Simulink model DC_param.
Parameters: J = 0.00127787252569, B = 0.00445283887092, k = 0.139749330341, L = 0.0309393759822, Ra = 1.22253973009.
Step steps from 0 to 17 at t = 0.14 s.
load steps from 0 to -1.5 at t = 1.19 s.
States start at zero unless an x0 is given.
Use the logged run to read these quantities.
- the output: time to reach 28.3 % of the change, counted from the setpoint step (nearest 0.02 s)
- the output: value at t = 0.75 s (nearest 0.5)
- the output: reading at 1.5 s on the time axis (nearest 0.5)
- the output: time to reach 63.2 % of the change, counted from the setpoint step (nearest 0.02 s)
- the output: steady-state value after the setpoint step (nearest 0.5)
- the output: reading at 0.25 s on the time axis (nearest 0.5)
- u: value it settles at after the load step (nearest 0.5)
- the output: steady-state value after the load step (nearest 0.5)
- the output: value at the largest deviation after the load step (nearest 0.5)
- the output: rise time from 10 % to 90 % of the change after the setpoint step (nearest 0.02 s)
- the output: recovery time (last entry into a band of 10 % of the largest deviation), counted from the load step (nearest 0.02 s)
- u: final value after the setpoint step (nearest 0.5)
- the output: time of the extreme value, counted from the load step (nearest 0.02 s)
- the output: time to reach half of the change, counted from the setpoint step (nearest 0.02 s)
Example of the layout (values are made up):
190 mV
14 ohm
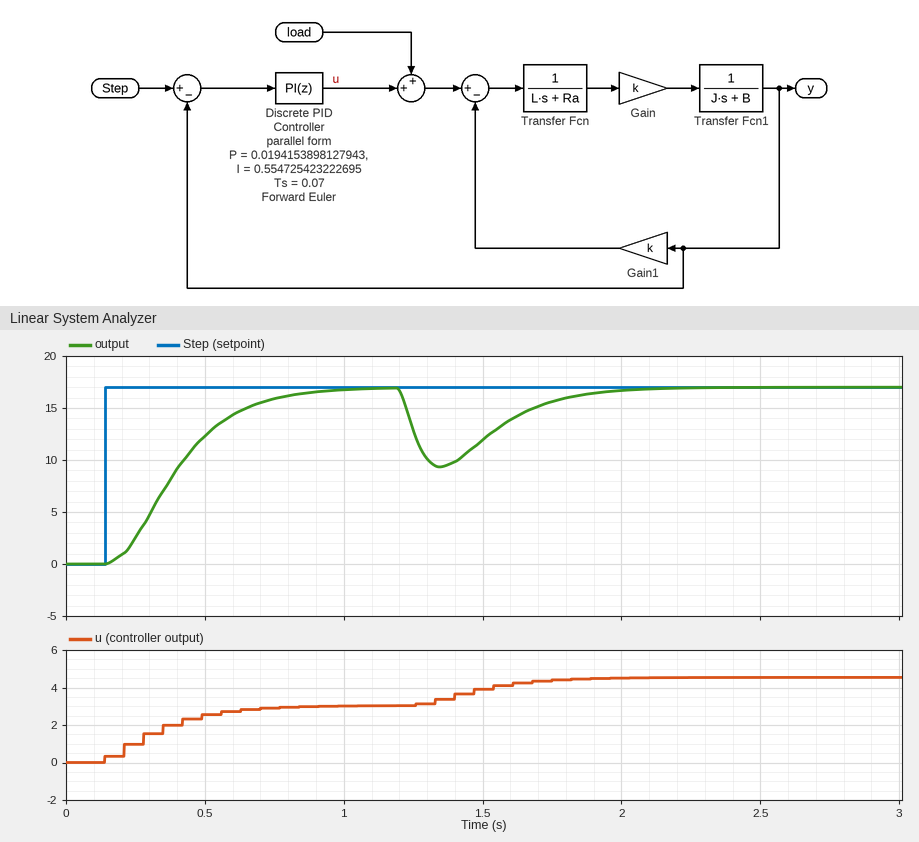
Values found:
0.16 s
16.0
12.0
0.30 s
17.0
2.5
4.5
17.0
9.5
0.44 s
0.66 s
3.0
0.16 s
0.24 s
